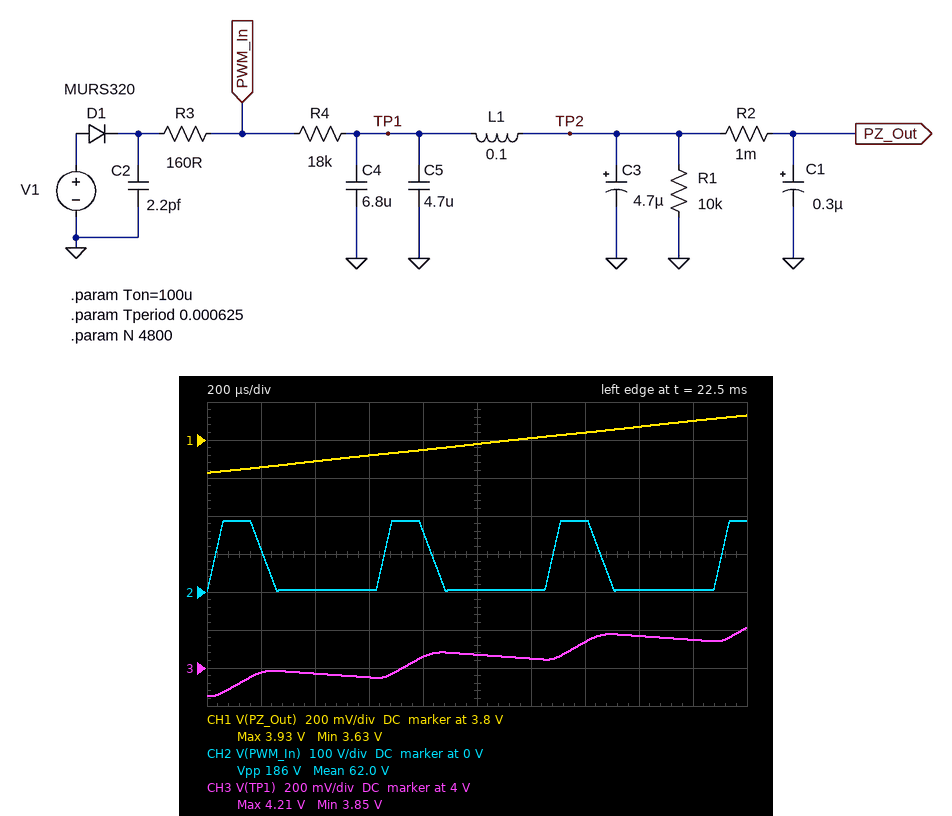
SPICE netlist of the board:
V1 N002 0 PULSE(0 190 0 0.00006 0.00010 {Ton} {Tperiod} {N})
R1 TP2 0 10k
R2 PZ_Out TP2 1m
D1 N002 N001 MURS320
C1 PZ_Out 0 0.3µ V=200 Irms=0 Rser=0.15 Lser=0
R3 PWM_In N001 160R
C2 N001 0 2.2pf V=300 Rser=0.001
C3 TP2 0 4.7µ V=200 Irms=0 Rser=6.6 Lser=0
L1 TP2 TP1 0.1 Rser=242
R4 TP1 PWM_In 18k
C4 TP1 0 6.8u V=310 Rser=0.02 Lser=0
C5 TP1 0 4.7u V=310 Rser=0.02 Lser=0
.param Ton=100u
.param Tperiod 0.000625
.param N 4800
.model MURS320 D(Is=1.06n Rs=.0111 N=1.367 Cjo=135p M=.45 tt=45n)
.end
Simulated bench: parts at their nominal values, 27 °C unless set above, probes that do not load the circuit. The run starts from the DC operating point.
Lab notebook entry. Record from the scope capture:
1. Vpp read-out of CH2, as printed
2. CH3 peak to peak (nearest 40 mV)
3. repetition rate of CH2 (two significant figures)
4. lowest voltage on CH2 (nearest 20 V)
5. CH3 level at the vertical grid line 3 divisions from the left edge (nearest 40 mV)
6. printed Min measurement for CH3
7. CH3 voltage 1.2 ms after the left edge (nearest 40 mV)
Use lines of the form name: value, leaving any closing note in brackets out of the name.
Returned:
Vpp read-out of CH2, as printed: 186 V
CH3 peak to peak: 360 mV
repetition rate of CH2: 1.6 kHz
lowest voltage on CH2: 0 V
CH3 level at the vertical grid line 3 divisions from the left edge: 3.96 V
printed Min measurement for CH3: 3.85 V
CH3 voltage 1.2 ms after the left edge: 4.04 V
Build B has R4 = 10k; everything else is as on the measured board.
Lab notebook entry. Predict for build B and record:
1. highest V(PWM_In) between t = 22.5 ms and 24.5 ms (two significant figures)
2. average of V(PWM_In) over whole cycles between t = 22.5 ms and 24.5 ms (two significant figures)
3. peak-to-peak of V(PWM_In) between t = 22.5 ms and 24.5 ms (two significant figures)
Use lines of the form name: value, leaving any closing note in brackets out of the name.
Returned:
highest V(PWM_In) between t = 22.5 ms and 24.5 ms: 190 V
average of V(PWM_In) over whole cycles between t = 22.5 ms and 24.5 ms: 58 V
peak-to-peak of V(PWM_In) between t = 22.5 ms and 24.5 ms: 180 V
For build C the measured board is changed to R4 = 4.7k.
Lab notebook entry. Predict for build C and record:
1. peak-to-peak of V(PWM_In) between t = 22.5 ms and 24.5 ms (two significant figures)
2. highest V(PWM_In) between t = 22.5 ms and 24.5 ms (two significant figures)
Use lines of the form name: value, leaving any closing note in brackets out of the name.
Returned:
peak-to-peak of V(PWM_In) between t = 22.5 ms and 24.5 ms: 170 V
highest V(PWM_In) between t = 22.5 ms and 24.5 ms: 180 V
